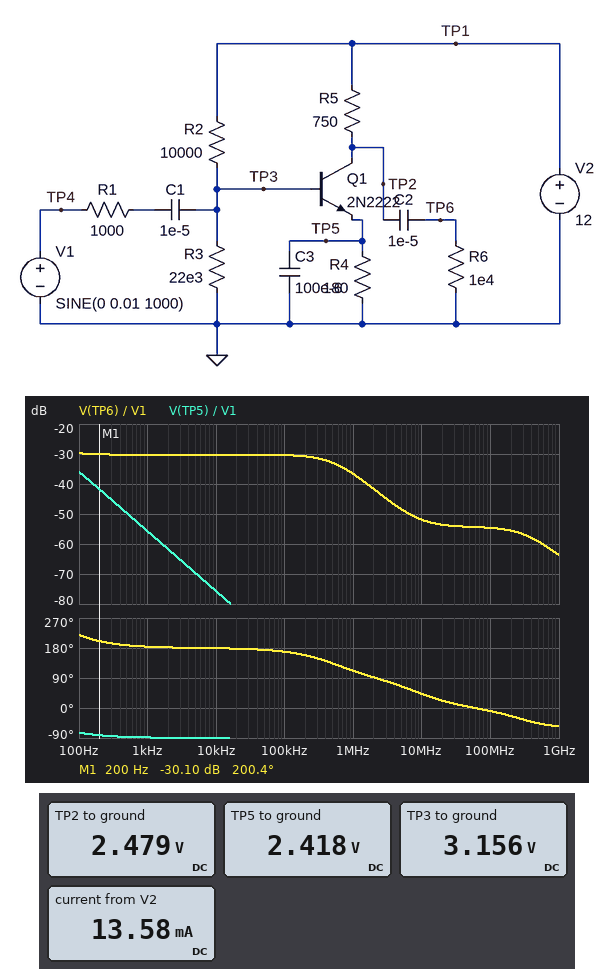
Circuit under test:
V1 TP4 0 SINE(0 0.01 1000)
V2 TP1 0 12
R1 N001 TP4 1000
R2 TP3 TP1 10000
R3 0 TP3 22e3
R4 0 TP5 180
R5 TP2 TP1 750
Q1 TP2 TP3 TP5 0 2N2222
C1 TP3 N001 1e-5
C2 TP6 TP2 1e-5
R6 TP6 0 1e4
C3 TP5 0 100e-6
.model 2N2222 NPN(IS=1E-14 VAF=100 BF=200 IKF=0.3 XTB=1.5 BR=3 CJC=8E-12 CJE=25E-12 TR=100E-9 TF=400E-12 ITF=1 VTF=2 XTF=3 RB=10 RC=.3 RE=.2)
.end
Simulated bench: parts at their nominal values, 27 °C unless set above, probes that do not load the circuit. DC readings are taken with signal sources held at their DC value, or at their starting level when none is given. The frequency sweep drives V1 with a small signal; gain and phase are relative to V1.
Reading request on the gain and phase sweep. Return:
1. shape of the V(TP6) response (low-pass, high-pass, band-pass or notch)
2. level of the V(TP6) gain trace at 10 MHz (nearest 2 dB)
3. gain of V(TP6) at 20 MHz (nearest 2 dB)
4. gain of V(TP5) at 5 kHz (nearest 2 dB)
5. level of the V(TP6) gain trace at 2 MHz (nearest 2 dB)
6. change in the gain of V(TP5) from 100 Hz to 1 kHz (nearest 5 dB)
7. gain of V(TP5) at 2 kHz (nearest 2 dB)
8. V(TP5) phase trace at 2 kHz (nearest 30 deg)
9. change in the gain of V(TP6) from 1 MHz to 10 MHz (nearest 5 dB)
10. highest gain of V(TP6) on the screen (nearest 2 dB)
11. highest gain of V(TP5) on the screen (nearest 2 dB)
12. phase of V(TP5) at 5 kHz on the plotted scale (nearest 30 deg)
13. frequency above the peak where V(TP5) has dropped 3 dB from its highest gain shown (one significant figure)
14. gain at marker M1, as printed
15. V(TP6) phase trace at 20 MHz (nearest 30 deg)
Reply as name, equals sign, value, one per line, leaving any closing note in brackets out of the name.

shape of the V(TP6) response = low-pass
level of the V(TP6) gain trace at 10 MHz = -52 dB
gain of V(TP6) at 20 MHz = -54 dB
gain of V(TP5) at 5 kHz = -70 dB
level of the V(TP6) gain trace at 2 MHz = -42 dB
change in the gain of V(TP5) from 100 Hz to 1 kHz = -20 dB
gain of V(TP5) at 2 kHz = -62 dB
V(TP5) phase trace at 2 kHz = -90 deg
change in the gain of V(TP6) from 1 MHz to 10 MHz = -15 dB
highest gain of V(TP6) on the screen = -30 dB
highest gain of V(TP5) on the screen = -36 dB
phase of V(TP5) at 5 kHz on the plotted scale = -90 deg
frequency above the peak where V(TP5) has dropped 3 dB from its highest gain shown = 100 Hz
gain at marker M1, as printed = -30.10 dB
V(TP6) phase trace at 20 MHz = 30 deg
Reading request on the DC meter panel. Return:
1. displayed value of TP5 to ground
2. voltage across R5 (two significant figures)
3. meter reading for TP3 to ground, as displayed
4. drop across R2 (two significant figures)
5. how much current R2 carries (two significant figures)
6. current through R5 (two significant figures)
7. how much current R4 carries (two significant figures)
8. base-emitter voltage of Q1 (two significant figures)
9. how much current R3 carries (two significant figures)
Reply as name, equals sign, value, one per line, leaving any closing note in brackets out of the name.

displayed value of TP5 to ground = 2.418 V
voltage across R5 = 9.5 V
meter reading for TP3 to ground, as displayed = 3.156 V
drop across R2 = 8.8 V
how much current R2 carries = 880 µA
current through R5 = 13 mA
how much current R4 carries = 13 mA
base-emitter voltage of Q1 = 740 mV
how much current R3 carries = 140 µA
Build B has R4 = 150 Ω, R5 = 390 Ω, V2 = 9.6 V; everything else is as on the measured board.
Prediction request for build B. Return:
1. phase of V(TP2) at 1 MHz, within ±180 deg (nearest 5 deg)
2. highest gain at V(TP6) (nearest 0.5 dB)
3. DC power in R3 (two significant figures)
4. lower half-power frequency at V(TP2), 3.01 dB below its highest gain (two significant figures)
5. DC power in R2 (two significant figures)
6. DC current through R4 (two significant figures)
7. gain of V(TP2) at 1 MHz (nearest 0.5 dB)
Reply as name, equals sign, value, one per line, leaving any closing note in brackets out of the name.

phase of V(TP2) at 1 MHz, within ±180 deg = 115 deg
highest gain at V(TP6) = -24.0 dB
DC power in R3 = 540 µW
lower half-power frequency at V(TP2), 3.01 dB below its highest gain = 19 Hz
DC power in R2 = 3.8 mW
DC current through R4 = 18 mA
gain of V(TP2) at 1 MHz = -30.5 dB
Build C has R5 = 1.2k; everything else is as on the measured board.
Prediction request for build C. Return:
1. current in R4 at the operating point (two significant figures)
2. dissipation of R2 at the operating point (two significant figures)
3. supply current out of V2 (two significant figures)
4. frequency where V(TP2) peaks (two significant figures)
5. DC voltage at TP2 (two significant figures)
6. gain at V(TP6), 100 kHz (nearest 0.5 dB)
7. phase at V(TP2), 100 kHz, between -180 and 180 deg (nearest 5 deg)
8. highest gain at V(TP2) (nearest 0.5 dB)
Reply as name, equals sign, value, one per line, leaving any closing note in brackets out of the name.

current in R4 at the operating point = 9.4 mA
dissipation of R2 at the operating point = 9.2 mW
supply current out of V2 = 9.5 mA
frequency where V(TP2) peaks = 14 Hz
DC voltage at TP2 = 1.7 V
gain at V(TP6), 100 kHz = -33.0 dB
phase at V(TP2), 100 kHz, between -180 and 180 deg = 170 deg
highest gain at V(TP2) = -26.0 dB
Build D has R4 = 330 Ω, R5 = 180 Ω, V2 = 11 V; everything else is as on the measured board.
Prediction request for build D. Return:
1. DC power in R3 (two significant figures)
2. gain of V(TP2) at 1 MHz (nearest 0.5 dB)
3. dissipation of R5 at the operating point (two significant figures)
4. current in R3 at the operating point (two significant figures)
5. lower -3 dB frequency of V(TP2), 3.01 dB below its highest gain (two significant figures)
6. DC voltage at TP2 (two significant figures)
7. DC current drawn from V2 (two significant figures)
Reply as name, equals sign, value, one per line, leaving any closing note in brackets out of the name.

DC power in R3 = 2.2 mW
gain of V(TP2) at 1 MHz = 23.0 dB
dissipation of R5 at the operating point = 62 mW
current in R3 at the operating point = 310 µA
lower -3 dB frequency of V(TP2), 3.01 dB below its highest gain = 250 Hz
DC voltage at TP2 = 7.7 V
DC current drawn from V2 = 19 mA
